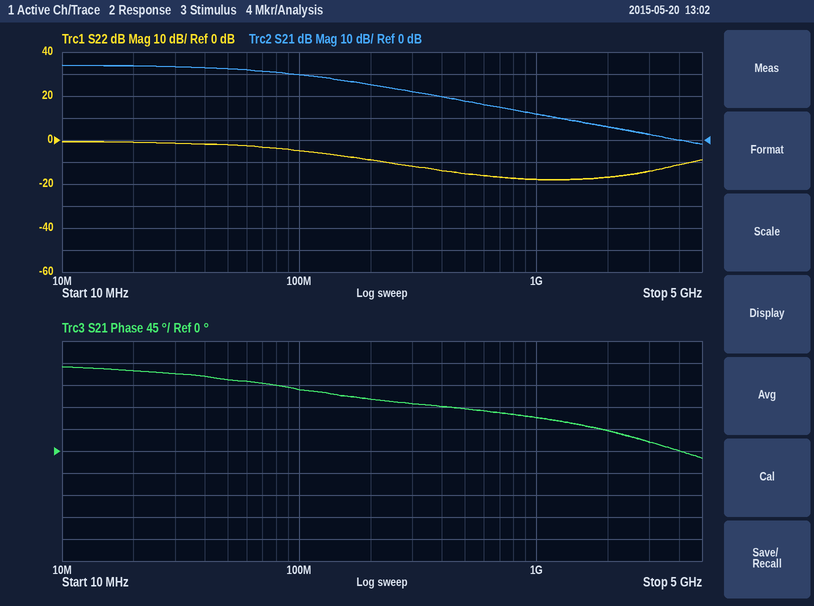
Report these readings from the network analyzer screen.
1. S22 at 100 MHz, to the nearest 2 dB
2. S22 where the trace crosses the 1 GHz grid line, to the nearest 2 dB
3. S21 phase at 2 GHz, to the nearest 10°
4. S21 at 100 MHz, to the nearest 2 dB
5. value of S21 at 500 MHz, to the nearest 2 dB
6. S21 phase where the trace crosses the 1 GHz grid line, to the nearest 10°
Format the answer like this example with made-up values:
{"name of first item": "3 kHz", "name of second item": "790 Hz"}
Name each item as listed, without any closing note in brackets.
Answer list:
{"S22 at 100 MHz, to the nearest 2 dB": "-4 dB", "S22 where the trace crosses the 1 GHz grid line, to the nearest 2 dB": "-18 dB", "S21 phase at 2 GHz, to the nearest 10°": "40°", "S21 at 100 MHz, to the nearest 2 dB": "30 dB", "value of S21 at 500 MHz, to the nearest 2 dB": "18 dB", "S21 phase where the trace crosses the 1 GHz grid line, to the nearest 10°": "70°"}
